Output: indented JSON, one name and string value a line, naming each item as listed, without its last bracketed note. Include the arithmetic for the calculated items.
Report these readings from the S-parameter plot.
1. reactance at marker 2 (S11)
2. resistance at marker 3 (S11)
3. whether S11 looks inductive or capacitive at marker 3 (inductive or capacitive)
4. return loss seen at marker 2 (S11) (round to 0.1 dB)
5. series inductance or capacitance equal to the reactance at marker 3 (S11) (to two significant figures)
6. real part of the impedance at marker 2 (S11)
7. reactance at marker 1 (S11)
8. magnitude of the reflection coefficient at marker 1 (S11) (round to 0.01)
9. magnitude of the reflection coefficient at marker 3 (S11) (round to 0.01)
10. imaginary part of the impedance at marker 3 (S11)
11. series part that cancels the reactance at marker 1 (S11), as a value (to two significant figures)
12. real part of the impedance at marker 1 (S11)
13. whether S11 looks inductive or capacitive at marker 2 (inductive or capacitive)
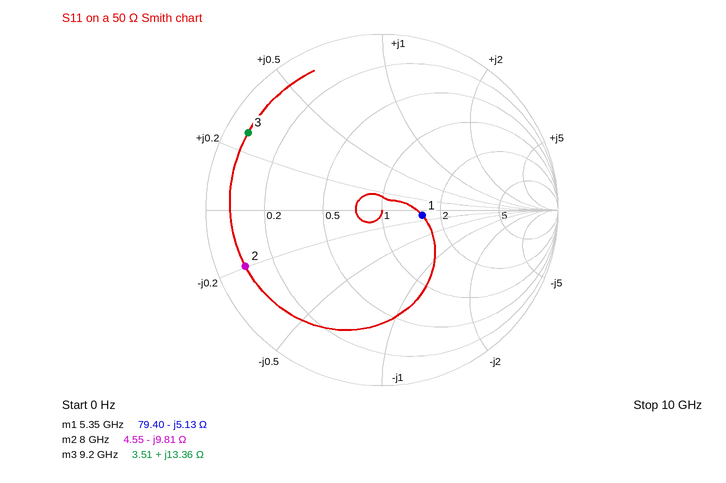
{
  "reactance at marker 2": "-9.81 Ω",
  "resistance at marker 3": "3.51 Ω",
  "whether S11 looks inductive or capacitive at marker 3": "inductive",
  "return loss seen at marker 2 (S11)": "1.5 dB",
  "series inductance or capacitance equal to the reactance at marker 3 (S11)": "L = 13.36 Ω/(2π × 9.2 GHz) ≈ 231 pH, so 230 pH to two significant figures",
  "real part of the impedance at marker 2": "4.55 Ω",
  "reactance at marker 1": "-5.13 Ω",
  "magnitude of the reflection coefficient at marker 1 (S11)": "0.23",
  "magnitude of the reflection coefficient at marker 3 (S11)": "0.88",
  "imaginary part of the impedance at marker 3": "+13.36 Ω",
  "series part that cancels the reactance at marker 1 (S11), as a value": "L = 5.13 Ω/(2π × 5.35 GHz) ≈ 153 pH, so 150 pH to two significant figures",
  "real part of the impedance at marker 1": "79.40 Ω",
  "whether S11 looks inductive or capacitive at marker 2": "capacitive"
}
